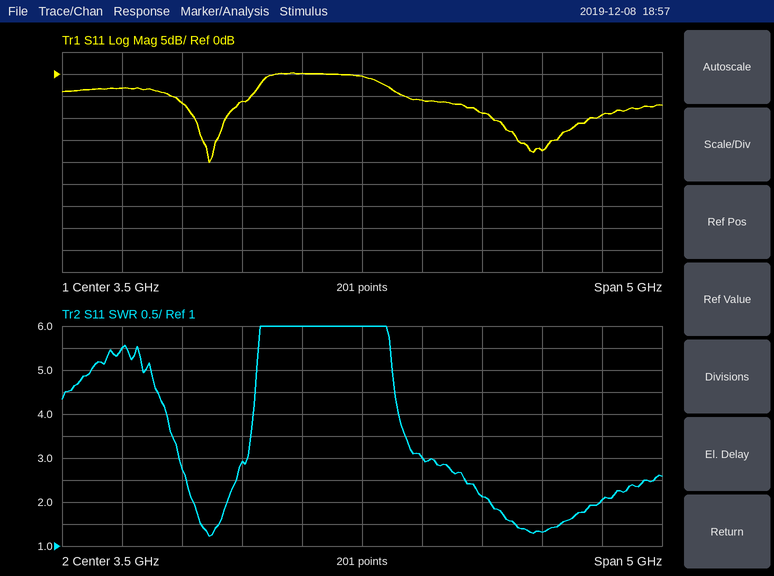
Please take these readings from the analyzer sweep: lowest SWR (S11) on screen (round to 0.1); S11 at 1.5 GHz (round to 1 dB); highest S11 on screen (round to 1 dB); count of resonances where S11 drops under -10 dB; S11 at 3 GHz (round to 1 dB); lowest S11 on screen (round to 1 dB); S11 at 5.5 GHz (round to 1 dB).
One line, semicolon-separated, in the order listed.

1.2; -3 dB; 0 dB; 2; 0 dB; -20 dB; -9 dB
